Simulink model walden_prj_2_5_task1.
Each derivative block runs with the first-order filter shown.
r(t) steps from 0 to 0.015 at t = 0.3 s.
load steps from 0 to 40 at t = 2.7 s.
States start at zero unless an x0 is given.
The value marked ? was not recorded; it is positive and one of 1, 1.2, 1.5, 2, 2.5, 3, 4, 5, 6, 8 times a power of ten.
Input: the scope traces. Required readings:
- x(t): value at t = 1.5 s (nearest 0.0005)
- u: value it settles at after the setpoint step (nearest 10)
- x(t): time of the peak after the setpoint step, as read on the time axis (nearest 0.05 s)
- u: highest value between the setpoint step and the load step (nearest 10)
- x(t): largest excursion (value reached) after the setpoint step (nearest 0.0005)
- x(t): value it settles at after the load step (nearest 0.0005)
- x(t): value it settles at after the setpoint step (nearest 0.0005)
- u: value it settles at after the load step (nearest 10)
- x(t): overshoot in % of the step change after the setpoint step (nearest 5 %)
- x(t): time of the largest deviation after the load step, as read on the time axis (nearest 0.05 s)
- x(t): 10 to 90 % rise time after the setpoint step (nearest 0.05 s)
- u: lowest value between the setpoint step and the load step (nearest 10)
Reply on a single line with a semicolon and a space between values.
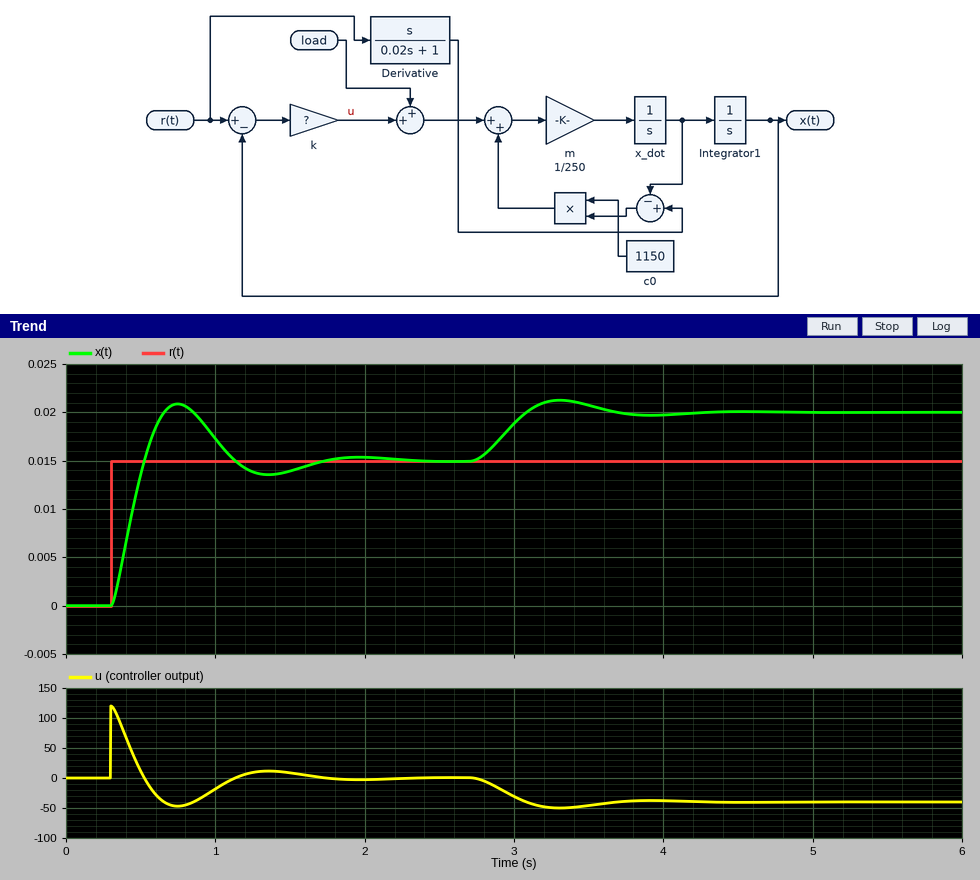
0.0140; 0; 0.75 s; 120; 0.0210; 0.0200; 0.0150; -40; 40 %; 3.30 s; 0.15 s; -50
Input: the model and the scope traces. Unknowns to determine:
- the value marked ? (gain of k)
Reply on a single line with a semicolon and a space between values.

8000
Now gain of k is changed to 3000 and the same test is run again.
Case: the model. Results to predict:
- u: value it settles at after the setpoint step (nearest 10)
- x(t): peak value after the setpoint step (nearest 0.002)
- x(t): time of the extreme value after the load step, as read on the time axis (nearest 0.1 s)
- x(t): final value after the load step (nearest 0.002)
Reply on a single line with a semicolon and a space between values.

0; 0.018; 3.9 s; 0.028
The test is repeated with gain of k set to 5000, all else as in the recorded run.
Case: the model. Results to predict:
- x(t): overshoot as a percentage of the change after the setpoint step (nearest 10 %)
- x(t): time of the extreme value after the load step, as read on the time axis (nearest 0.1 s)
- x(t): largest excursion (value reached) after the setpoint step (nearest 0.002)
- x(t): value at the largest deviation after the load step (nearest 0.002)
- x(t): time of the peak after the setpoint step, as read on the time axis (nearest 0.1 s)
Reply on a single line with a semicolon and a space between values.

30 %; 3.5 s; 0.020; 0.024; 0.8 s
